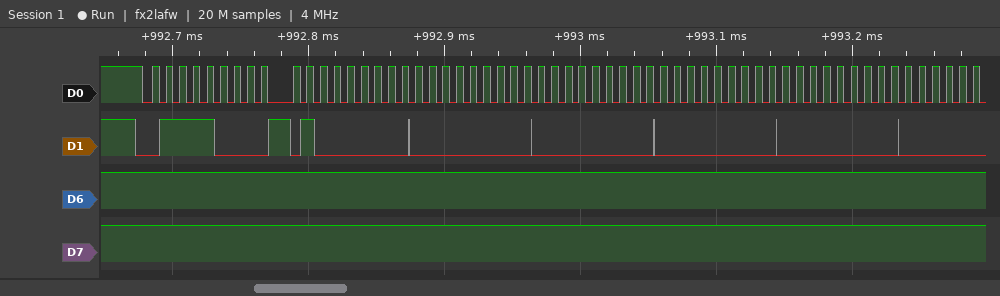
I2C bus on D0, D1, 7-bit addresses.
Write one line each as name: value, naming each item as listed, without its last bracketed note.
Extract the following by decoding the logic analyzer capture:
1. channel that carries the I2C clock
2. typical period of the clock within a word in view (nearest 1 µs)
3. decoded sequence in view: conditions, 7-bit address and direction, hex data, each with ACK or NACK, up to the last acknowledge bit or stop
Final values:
channel that carries the I2C clock: D0
typical period of the clock within a word in view: 10 µs
decoded sequence in view: conditions, 7-bit address and direction, hex data, each with ACK or NACK, up to the last acknowledge bit or stop: start, address 3C write ACK, 40 ACK, 00 ACK, 00 ACK, 00 ACK, 00 ACK
